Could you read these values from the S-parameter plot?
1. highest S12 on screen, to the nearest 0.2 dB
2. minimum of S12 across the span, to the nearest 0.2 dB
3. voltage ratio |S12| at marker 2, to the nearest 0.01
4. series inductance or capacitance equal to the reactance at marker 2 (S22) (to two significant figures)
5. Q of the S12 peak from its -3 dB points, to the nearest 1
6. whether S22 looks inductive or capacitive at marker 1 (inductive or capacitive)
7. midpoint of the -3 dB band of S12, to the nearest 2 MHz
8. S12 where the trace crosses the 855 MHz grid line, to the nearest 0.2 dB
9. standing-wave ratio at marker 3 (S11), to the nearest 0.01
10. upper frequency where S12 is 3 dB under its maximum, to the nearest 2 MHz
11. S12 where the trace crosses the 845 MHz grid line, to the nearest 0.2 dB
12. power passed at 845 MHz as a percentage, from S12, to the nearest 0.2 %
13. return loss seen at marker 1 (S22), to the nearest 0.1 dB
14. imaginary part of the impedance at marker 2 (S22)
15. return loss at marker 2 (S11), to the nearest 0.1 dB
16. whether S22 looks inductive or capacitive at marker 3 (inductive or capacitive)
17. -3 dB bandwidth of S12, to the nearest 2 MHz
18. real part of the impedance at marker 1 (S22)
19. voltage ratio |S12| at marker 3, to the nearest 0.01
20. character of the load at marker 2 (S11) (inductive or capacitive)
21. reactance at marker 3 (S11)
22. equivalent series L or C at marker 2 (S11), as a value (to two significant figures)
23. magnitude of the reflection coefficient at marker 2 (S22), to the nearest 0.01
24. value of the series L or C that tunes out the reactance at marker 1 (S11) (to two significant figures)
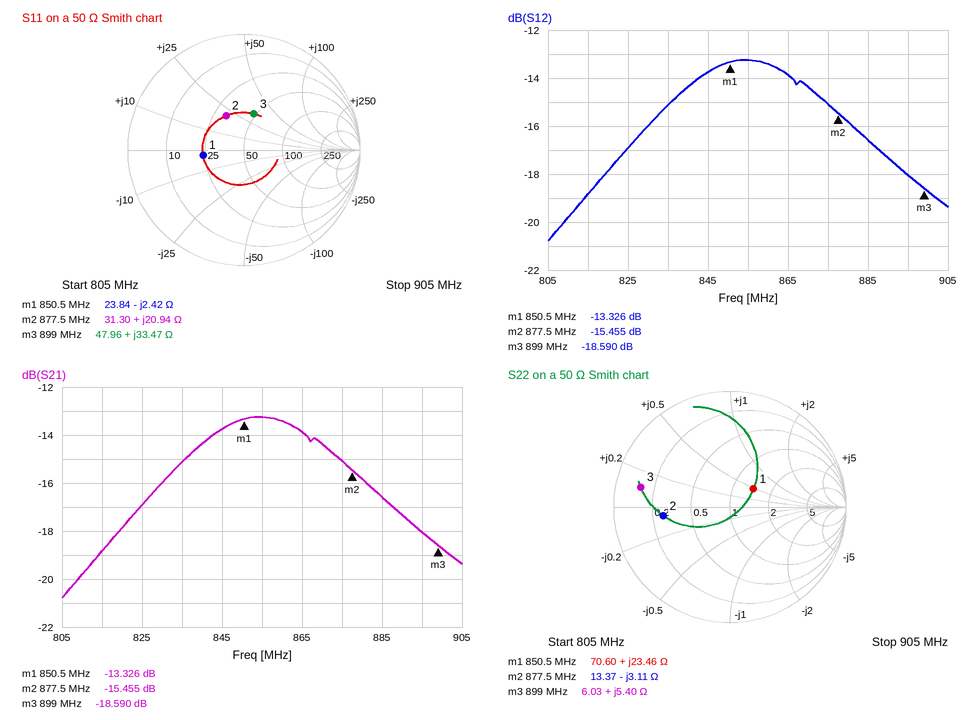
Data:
-13.2 dB
-20.8 dB
0.17
58 pF
16
inductive
856 MHz
-13.2 dB
1.96
882 MHz
-13.8 dB
4.2 %
11.9 dB
-3.11 Ω
9.5 dB
inductive
54 MHz
70.60 Ω
0.12
inductive
+33.47 Ω
3.8 nH
0.58
450 pH
